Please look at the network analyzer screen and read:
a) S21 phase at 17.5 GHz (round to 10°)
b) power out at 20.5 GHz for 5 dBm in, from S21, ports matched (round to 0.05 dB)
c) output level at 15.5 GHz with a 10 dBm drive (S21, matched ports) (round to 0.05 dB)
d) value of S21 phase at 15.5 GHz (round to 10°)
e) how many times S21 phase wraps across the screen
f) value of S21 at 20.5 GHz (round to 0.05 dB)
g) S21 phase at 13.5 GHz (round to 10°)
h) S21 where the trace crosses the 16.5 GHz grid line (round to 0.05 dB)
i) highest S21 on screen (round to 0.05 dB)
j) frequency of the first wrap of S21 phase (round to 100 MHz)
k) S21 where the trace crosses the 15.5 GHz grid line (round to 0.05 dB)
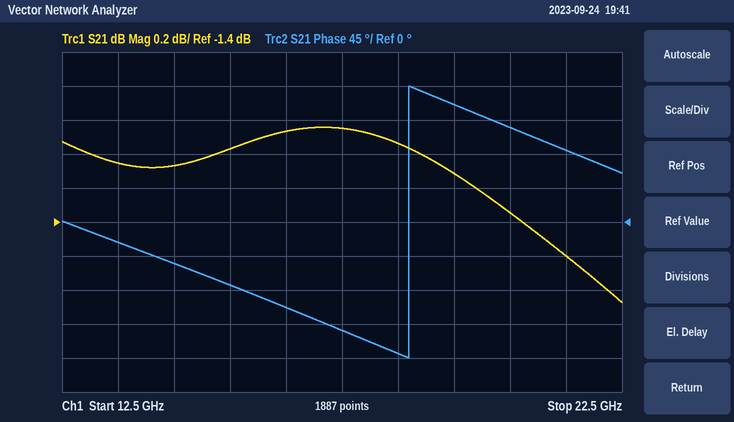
-140°
3.65 dBm
9.05 dBm
-80°
1
-1.35 dB
-30°
-0.85 dB
-0.85 dB
18.7 GHz
-0.95 dB
